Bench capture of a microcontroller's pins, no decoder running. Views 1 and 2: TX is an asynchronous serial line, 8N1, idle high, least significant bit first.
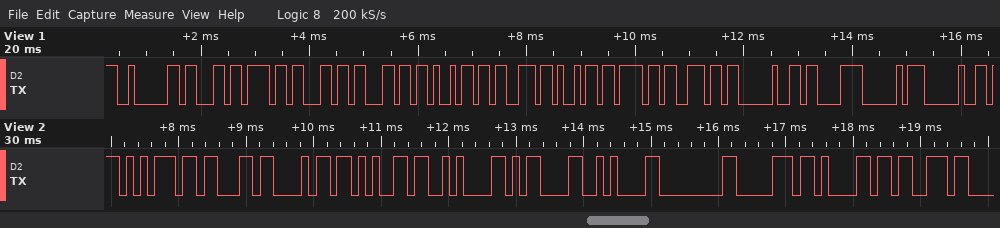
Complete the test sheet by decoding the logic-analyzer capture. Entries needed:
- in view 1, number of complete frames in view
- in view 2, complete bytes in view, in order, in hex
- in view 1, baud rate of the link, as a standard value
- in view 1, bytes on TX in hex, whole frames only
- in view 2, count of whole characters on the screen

14
75 63 68 65 0A 0D 0A 00 70 61 73
9600 baud
02 63 6F 6C 6C 69 73 69 6F 6E 20 C3 A0 20
11
